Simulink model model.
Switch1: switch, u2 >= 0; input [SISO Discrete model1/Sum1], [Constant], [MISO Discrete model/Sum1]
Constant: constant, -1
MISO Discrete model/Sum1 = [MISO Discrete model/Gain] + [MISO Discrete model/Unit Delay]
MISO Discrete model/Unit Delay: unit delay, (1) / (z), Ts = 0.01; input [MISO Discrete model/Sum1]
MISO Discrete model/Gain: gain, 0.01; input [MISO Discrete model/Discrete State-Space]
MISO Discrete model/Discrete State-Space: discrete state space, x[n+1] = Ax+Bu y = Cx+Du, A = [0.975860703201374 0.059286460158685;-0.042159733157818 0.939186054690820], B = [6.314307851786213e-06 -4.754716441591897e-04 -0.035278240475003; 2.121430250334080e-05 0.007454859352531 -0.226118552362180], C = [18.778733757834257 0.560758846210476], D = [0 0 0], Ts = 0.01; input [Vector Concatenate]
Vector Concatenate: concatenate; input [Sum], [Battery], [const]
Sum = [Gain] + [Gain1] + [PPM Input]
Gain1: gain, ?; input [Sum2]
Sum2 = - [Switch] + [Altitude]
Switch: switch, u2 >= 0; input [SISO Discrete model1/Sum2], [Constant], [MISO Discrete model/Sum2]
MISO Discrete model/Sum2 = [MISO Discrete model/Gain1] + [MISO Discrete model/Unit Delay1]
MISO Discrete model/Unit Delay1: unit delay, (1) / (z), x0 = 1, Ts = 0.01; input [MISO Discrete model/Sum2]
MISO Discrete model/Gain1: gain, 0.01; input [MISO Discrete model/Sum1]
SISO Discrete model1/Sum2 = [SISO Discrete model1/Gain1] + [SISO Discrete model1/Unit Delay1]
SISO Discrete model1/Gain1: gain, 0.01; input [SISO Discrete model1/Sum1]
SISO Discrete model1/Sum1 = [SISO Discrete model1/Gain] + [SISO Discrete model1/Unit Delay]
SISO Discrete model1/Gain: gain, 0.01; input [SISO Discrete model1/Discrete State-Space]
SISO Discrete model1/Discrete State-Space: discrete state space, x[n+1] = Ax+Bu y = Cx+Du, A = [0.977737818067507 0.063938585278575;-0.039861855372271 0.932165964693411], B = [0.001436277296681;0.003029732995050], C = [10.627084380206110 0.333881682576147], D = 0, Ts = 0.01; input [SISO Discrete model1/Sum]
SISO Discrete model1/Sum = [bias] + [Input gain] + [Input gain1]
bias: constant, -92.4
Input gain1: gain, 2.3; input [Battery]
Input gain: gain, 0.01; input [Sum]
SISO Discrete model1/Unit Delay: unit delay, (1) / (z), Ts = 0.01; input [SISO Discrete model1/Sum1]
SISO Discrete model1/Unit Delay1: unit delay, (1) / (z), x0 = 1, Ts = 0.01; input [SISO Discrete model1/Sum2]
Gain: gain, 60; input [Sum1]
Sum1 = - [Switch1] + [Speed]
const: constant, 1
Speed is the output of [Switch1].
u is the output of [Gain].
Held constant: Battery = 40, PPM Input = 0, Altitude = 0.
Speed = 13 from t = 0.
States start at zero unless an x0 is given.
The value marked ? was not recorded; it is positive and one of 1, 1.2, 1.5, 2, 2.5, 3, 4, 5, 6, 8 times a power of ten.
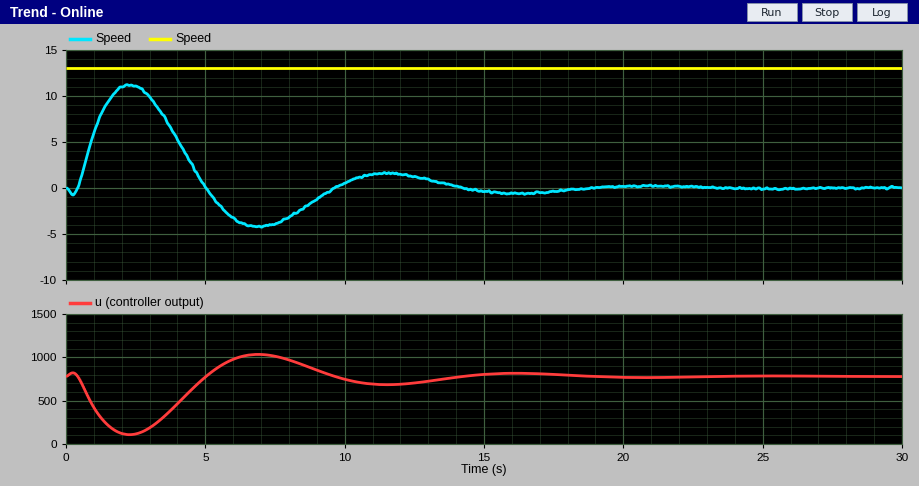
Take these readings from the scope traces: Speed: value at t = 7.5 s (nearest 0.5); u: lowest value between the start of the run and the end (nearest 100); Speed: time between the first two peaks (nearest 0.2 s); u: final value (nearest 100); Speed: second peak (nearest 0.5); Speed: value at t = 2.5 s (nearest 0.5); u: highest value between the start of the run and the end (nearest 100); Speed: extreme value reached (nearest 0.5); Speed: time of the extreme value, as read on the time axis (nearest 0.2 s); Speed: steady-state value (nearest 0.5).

-4.0
100
9.2 s
800
1.5
11.0
1000
11.0
2.2 s
0.0
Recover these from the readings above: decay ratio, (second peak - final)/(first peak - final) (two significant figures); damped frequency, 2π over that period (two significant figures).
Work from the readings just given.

0.14
0.68 rad/s
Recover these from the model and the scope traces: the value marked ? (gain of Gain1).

60
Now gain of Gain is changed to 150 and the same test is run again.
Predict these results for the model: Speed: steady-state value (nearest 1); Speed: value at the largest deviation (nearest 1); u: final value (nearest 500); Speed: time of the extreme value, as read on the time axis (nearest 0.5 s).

0
13
2000
1.5 s
